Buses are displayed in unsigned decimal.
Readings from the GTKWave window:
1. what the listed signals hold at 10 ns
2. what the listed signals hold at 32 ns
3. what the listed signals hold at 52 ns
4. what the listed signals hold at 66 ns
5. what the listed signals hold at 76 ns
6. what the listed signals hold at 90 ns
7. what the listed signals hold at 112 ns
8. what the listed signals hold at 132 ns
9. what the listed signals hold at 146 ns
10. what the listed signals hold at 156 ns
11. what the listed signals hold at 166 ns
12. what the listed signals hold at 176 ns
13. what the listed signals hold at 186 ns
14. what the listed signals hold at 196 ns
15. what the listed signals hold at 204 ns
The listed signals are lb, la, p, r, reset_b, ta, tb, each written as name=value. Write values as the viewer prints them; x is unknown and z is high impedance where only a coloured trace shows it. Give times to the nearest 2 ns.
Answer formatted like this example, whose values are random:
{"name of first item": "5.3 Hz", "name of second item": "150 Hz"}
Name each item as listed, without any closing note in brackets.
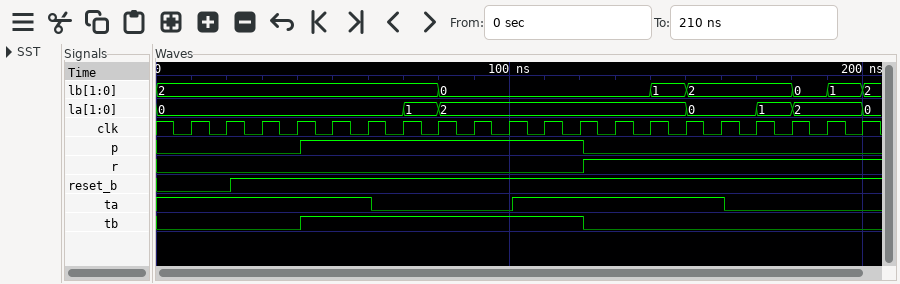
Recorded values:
{"what the listed signals hold at 10 ns": "lb=2, la=0, p=0, r=0, reset_b=0, ta=1, tb=0", "what the listed signals hold at 32 ns": "lb=2, la=0, p=0, r=0, reset_b=1, ta=1, tb=0", "what the listed signals hold at 52 ns": "lb=2, la=0, p=1, r=0, reset_b=1, ta=1, tb=1", "what the listed signals hold at 66 ns": "lb=2, la=0, p=1, r=0, reset_b=1, ta=0, tb=1", "what the listed signals hold at 76 ns": "lb=2, la=1, p=1, r=0, reset_b=1, ta=0, tb=1", "what the listed signals hold at 90 ns": "lb=0, la=2, p=1, r=0, reset_b=1, ta=0, tb=1", "what the listed signals hold at 112 ns": "lb=0, la=2, p=1, r=0, reset_b=1, ta=1, tb=1", "what the listed signals hold at 132 ns": "lb=0, la=2, p=0, r=1, reset_b=1, ta=1, tb=0", "what the listed signals hold at 146 ns": "lb=1, la=2, p=0, r=1, reset_b=1, ta=1, tb=0", "what the listed signals hold at 156 ns": "lb=2, la=0, p=0, r=1, reset_b=1, ta=1, tb=0", "what the listed signals hold at 166 ns": "lb=2, la=0, p=0, r=1, reset_b=1, ta=0, tb=0", "what the listed signals hold at 176 ns": "lb=2, la=1, p=0, r=1, reset_b=1, ta=0, tb=0", "what the listed signals hold at 186 ns": "lb=0, la=2, p=0, r=1, reset_b=1, ta=0, tb=0", "what the listed signals hold at 196 ns": "lb=1, la=2, p=0, r=1, reset_b=1, ta=0, tb=0", "what the listed signals hold at 204 ns": "lb=2, la=0, p=0, r=1, reset_b=1, ta=0, tb=0"}
